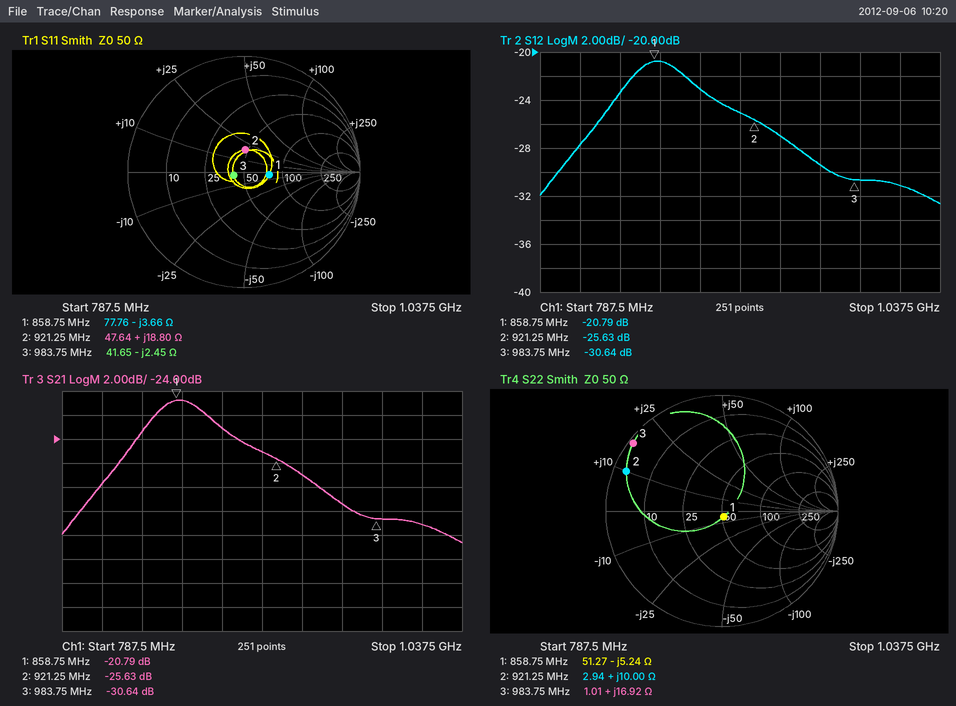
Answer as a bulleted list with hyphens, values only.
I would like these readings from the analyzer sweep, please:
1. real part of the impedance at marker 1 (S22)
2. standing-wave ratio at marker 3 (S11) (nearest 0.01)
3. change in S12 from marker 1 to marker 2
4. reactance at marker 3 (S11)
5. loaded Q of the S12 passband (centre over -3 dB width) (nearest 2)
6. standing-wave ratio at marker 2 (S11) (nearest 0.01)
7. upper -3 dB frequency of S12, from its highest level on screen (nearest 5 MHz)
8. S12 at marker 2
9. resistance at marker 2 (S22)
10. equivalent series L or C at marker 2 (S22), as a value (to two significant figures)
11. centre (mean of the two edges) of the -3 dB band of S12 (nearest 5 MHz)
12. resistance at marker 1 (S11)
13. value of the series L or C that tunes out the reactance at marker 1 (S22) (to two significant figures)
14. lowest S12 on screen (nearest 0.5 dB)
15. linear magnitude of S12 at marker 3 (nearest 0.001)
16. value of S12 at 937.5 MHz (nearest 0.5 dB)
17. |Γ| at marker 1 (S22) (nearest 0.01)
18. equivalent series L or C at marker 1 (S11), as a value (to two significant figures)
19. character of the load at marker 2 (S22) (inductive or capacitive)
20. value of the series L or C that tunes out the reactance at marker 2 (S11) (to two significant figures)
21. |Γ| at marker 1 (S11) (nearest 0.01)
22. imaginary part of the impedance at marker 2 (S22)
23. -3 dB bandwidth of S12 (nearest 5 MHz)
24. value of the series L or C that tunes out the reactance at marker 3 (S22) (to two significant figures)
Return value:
- 51.27 Ω
- 1.21
- -4.84 dB
- -2.45 Ω
- 14
- 1.47
- 895 MHz
- -25.63 dB
- 2.94 Ω
- 1.7 nH
- 865 MHz
- 77.76 Ω
- 970 pH
- -32.5 dB
- 0.029
- -27.0 dB
- 0.05
- 51 pF
- inductive
- 9.2 pF
- 0.22
- +10.00 Ω
- 60 MHz
- 9.6 pF
